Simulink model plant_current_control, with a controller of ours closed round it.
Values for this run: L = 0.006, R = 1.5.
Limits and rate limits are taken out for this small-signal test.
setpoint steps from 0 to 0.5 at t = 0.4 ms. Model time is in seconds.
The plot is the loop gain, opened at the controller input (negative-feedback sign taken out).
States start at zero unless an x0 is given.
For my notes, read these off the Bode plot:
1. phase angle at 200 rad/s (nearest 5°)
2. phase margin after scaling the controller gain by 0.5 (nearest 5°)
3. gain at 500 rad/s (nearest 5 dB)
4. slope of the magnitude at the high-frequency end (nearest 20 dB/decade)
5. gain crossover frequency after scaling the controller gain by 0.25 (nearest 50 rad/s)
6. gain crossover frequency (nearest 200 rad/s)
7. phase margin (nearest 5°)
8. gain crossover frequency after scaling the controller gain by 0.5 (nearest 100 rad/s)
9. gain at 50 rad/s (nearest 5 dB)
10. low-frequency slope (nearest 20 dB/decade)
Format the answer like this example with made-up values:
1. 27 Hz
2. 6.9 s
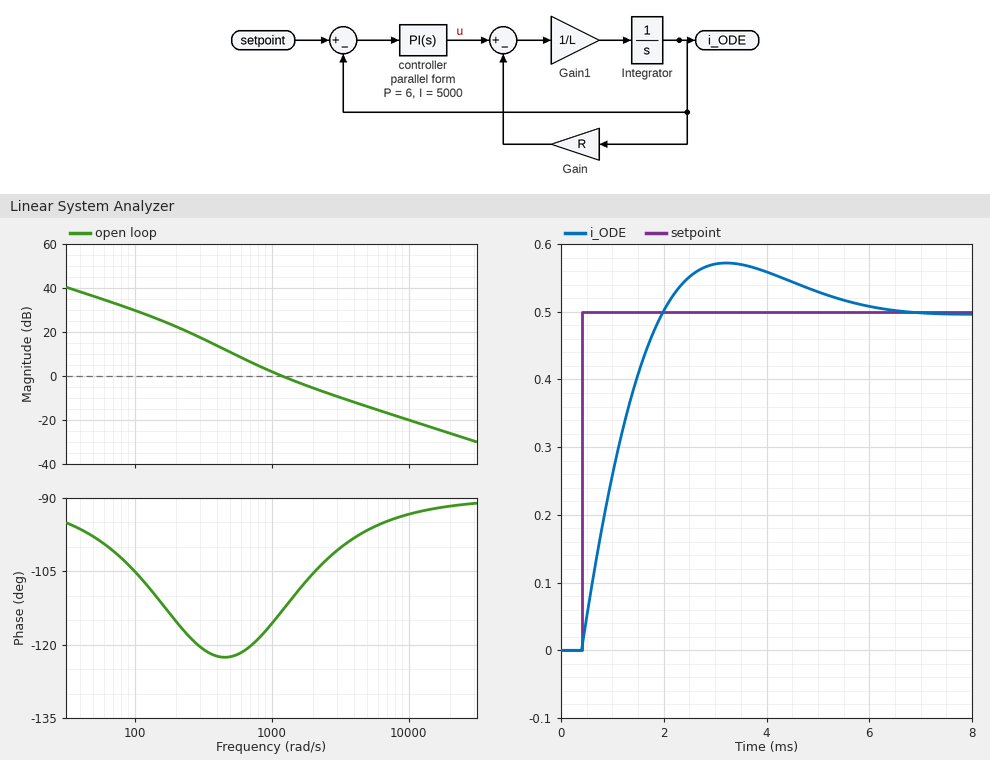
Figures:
1. -115°
2. 60°
3. 10 dB
4. -20 dB/decade
5. 450 rad/s
6. 1200 rad/s
7. 65°
8. 700 rad/s
9. 35 dB
10. -20 dB/decade
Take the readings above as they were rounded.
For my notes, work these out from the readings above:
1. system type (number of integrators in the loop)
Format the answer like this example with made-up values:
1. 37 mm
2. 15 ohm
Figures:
1. 1
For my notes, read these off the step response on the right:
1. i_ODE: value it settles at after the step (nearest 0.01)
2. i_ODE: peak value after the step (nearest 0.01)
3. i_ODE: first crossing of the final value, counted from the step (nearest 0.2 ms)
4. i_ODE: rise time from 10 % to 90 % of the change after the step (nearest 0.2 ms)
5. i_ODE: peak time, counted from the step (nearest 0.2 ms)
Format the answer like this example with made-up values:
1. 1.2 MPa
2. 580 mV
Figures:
1. 0.50
2. 0.57
3. 1.6 ms
4. 1.2 ms
5. 2.8 ms
